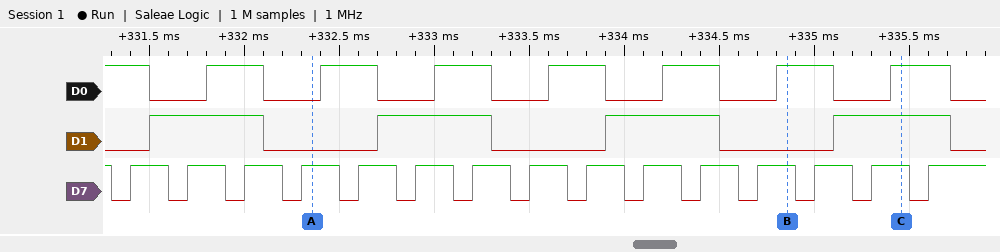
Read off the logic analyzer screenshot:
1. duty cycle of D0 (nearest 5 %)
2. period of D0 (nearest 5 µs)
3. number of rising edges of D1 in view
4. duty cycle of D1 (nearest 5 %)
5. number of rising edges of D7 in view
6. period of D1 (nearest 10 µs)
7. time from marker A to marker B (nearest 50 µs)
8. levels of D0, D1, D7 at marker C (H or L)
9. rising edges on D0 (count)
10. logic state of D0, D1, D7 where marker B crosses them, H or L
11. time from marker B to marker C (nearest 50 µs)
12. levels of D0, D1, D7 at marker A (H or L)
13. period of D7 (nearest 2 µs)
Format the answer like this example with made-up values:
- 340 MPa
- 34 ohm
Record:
- 50 %
- 600 µs
- 4
- 50 %
- 15
- 1200 µs
- 2500 µs
- D0=H, D1=H, D7=H
- 7
- D0=H, D1=L, D7=H
- 600 µs
- D0=L, D1=L, D7=H
- 300 µs
